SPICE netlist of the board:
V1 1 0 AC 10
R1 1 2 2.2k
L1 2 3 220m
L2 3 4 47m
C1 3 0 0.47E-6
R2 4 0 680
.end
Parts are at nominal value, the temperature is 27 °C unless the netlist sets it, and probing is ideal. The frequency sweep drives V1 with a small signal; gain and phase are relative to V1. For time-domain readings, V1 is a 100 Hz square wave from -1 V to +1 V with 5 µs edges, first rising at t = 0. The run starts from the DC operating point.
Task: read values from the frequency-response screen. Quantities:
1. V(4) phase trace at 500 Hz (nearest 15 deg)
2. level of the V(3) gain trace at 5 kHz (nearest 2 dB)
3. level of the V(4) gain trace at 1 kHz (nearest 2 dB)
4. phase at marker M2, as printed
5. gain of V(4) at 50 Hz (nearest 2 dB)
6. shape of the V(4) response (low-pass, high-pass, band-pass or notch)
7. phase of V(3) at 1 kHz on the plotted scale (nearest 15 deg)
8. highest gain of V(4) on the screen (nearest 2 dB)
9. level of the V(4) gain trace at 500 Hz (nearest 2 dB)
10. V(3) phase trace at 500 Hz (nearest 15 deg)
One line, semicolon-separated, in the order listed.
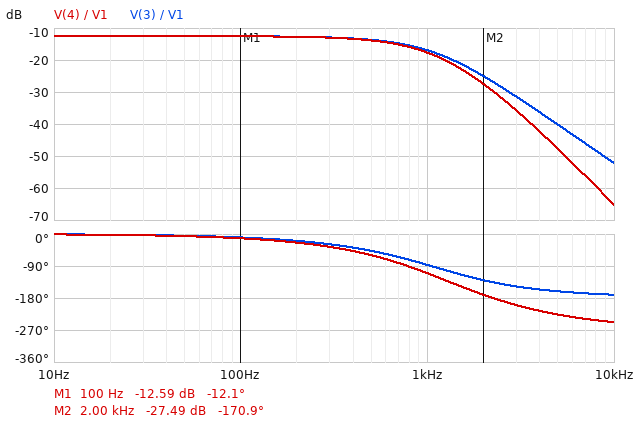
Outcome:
-60 deg; -40 dB; -18 dB; -170.9 deg; -12 dB; low-pass; -90 deg; -12 dB; -14 dB; -45 deg
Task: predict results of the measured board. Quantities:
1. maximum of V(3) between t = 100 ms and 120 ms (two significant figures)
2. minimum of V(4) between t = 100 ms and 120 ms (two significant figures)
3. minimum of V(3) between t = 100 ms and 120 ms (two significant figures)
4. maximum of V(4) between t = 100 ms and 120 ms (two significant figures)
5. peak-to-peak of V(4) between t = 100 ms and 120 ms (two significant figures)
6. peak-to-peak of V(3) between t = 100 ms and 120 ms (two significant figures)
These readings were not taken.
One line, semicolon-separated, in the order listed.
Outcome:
240 mV; -240 mV; -240 mV; 240 mV; 470 mV; 470 mV
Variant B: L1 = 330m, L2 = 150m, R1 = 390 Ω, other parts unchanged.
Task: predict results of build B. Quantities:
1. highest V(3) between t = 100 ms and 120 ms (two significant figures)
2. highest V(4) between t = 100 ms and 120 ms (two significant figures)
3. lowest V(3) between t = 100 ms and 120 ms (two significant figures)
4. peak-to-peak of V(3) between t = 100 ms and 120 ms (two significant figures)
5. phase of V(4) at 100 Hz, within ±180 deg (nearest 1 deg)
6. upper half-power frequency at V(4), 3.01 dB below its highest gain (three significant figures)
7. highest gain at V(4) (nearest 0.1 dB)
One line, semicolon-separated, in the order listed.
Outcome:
790 mV; 700 mV; -790 mV; 1.6 V; -20 deg; 668 Hz; -3.9 dB
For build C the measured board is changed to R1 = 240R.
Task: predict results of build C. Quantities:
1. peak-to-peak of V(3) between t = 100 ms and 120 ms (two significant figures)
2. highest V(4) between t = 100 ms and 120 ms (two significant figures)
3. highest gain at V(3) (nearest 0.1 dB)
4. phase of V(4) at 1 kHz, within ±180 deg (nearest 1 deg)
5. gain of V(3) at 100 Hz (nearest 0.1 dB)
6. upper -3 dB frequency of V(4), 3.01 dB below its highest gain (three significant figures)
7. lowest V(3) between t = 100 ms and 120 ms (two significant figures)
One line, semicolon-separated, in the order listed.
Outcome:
1.8 V; 870 mV; -2.3 dB; -155 deg; -2.6 dB; 718 Hz; -880 mV
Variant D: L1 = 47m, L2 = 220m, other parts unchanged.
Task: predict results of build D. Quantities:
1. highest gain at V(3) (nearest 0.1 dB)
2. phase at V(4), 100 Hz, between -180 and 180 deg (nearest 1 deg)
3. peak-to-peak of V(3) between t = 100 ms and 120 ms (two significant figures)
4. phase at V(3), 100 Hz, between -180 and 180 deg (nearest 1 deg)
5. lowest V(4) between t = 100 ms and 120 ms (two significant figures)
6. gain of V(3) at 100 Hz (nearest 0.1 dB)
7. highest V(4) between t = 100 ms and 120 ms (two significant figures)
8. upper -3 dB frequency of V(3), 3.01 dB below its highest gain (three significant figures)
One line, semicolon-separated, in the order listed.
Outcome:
-9.6 dB; -12 deg; 730 mV; -1 deg; -290 mV; -12.3 dB; 290 mV; 826 Hz
